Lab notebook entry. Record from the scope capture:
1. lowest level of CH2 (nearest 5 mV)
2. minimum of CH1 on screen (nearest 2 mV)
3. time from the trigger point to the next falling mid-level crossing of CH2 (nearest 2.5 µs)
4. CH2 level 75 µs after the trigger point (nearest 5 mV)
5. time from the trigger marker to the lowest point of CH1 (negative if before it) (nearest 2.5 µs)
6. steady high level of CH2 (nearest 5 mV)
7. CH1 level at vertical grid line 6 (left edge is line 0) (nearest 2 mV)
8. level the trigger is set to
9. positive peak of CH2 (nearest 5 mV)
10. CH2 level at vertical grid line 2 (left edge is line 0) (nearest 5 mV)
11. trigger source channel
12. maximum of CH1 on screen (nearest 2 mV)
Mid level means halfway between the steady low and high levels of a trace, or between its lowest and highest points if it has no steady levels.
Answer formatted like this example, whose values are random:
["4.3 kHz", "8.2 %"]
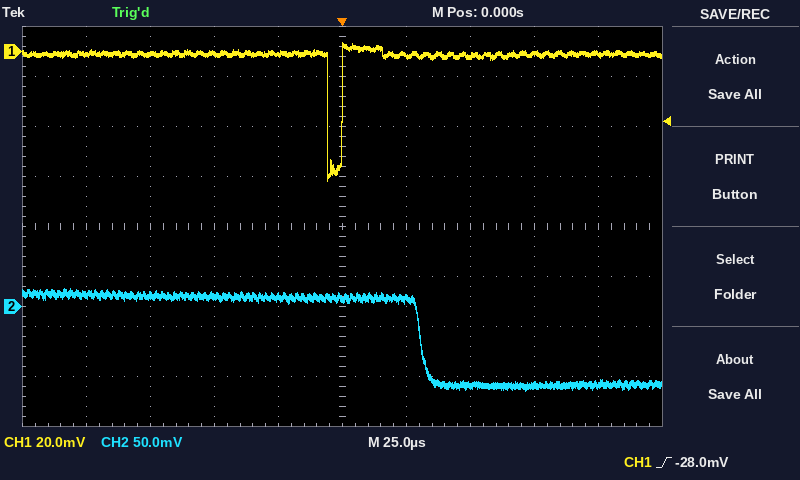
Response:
["-85 mV", "-52 mV", "30.0 µs", "-80 mV", "-5.0 µs", "10 mV", "-2 mV", "-28.0 mV", "20 mV", "10 mV", "CH1", "4 mV"]
